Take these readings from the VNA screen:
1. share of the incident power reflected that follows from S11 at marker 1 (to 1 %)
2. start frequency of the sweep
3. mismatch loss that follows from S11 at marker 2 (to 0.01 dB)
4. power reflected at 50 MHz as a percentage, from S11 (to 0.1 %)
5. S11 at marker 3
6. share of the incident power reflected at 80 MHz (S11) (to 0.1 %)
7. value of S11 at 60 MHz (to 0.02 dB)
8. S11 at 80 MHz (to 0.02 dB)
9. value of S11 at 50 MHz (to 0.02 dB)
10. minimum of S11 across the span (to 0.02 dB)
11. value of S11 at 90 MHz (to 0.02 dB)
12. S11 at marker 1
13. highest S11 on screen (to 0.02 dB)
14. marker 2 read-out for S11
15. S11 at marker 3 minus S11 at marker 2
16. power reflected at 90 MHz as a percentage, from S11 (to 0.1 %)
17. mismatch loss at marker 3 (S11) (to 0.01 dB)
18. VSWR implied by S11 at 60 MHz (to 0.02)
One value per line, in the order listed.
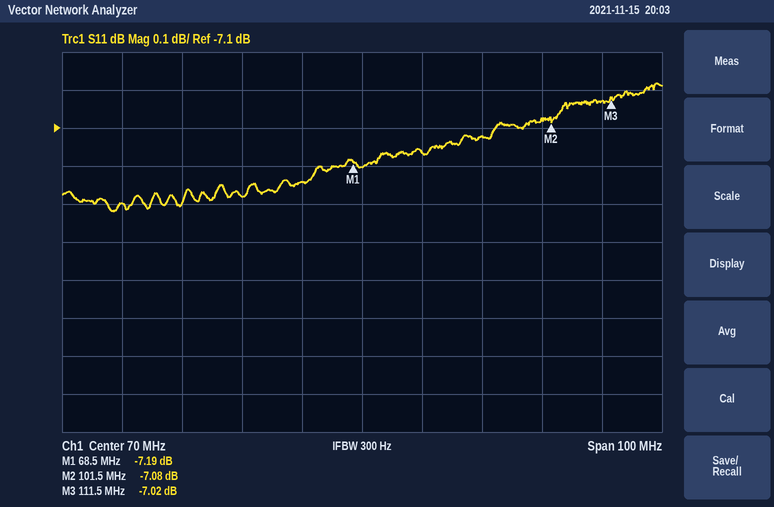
19 %
20 MHz
0.95 dB
18.7 %
-7.02 dB
19.2 %
-7.24 dB
-7.16 dB
-7.28 dB
-7.32 dB
-7.12 dB
-7.19 dB
-6.98 dB
-7.08 dB
0.06 dB
19.4 %
0.96 dB
2.54
